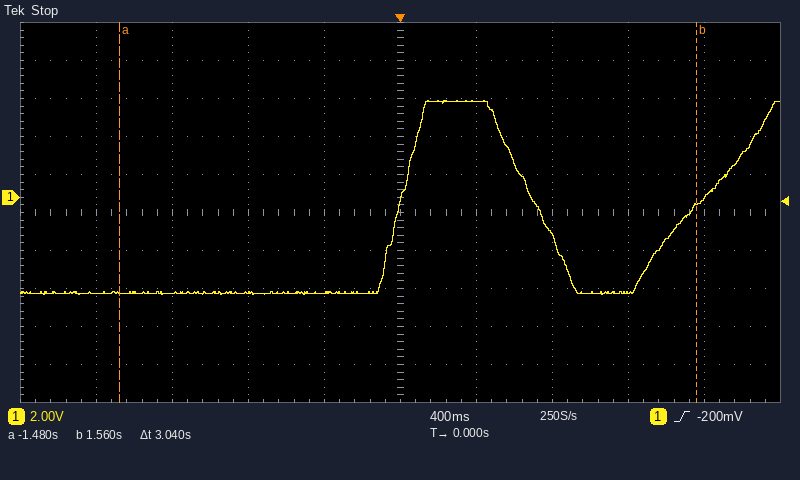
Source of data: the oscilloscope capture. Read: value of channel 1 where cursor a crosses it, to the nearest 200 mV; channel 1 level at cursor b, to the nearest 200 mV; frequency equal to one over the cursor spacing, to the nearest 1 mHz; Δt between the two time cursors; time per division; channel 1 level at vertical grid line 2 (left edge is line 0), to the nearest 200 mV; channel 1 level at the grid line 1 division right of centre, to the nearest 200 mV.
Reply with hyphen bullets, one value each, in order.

- -5.0 V
- -400 mV
- 329 mHz
- 3.04 s
- 400 ms
- -5.0 V
- 5.0 V
